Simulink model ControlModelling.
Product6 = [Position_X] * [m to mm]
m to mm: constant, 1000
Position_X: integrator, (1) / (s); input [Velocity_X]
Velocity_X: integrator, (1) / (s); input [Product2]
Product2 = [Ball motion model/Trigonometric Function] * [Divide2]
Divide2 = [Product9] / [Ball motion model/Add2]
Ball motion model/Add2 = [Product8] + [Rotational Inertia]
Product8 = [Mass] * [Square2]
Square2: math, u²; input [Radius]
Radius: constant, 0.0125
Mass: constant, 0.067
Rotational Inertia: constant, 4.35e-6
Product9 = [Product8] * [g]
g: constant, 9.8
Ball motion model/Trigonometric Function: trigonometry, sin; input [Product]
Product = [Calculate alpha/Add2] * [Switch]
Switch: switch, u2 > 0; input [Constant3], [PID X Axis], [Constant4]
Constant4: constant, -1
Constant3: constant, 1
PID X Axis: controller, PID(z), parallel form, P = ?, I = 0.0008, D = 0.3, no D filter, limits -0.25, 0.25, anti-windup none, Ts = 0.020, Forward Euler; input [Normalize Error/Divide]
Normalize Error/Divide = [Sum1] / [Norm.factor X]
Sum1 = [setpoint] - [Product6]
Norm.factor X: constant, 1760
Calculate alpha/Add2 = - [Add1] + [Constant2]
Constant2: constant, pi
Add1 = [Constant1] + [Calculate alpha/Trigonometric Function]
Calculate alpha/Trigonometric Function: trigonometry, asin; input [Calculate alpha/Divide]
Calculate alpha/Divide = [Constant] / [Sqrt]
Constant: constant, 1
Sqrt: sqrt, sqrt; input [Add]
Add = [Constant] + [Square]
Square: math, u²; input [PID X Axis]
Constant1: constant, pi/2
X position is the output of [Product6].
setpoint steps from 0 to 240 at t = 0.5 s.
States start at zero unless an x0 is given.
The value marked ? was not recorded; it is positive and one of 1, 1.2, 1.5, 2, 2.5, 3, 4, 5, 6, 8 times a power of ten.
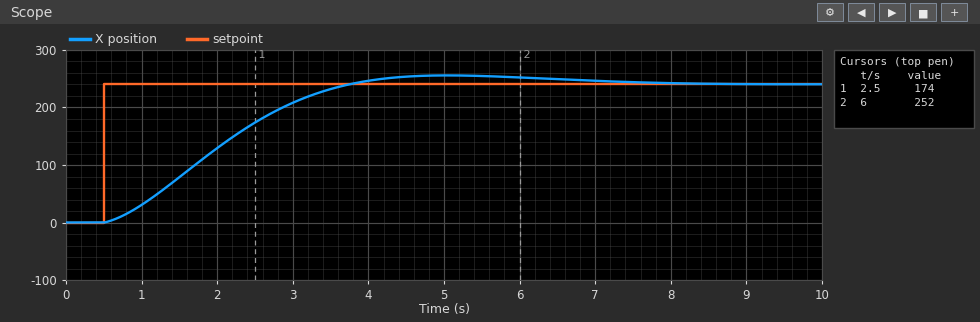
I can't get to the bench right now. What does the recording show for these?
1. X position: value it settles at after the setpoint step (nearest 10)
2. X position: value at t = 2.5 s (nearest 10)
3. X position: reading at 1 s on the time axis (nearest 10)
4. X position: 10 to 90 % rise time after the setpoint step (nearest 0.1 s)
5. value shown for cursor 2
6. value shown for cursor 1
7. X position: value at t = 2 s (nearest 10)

240
170
30
2.2 s
252
174
130
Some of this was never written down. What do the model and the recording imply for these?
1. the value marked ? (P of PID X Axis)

0.2
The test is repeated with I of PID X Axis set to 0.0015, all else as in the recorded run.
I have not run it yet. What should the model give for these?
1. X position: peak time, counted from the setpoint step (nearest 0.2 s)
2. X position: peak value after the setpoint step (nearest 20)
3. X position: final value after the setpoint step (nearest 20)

4.6 s
260
240
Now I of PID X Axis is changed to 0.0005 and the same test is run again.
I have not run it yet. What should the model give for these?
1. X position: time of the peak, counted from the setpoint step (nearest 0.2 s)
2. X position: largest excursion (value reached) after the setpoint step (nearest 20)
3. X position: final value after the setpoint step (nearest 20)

4.6 s
260
240
